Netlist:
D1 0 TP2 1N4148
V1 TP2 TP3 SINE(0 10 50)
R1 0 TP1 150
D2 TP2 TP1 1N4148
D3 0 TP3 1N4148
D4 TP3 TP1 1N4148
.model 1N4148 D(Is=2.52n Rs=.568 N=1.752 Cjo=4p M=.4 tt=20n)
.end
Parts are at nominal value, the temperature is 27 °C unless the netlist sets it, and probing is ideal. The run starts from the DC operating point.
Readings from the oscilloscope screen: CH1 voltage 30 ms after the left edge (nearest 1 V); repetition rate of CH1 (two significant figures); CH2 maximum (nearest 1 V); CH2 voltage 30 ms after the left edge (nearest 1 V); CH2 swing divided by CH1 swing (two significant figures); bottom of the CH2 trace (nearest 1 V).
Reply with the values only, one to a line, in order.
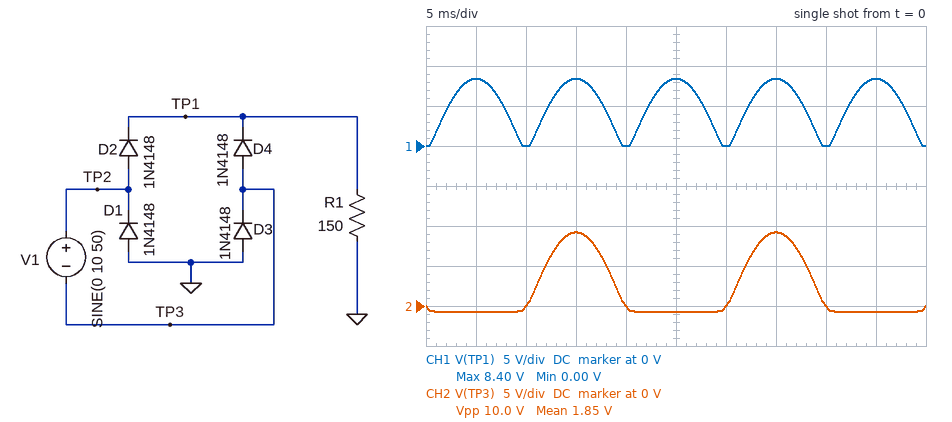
0 V
100 Hz
9 V
0 V
1.2
-1 V
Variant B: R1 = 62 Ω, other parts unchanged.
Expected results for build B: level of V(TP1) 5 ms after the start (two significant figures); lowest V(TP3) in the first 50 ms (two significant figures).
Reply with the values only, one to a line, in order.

8.2 V
-880 mV
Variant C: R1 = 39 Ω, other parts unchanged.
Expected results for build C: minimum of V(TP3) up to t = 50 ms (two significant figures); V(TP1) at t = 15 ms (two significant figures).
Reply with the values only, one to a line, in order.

-940 mV
8.1 V
